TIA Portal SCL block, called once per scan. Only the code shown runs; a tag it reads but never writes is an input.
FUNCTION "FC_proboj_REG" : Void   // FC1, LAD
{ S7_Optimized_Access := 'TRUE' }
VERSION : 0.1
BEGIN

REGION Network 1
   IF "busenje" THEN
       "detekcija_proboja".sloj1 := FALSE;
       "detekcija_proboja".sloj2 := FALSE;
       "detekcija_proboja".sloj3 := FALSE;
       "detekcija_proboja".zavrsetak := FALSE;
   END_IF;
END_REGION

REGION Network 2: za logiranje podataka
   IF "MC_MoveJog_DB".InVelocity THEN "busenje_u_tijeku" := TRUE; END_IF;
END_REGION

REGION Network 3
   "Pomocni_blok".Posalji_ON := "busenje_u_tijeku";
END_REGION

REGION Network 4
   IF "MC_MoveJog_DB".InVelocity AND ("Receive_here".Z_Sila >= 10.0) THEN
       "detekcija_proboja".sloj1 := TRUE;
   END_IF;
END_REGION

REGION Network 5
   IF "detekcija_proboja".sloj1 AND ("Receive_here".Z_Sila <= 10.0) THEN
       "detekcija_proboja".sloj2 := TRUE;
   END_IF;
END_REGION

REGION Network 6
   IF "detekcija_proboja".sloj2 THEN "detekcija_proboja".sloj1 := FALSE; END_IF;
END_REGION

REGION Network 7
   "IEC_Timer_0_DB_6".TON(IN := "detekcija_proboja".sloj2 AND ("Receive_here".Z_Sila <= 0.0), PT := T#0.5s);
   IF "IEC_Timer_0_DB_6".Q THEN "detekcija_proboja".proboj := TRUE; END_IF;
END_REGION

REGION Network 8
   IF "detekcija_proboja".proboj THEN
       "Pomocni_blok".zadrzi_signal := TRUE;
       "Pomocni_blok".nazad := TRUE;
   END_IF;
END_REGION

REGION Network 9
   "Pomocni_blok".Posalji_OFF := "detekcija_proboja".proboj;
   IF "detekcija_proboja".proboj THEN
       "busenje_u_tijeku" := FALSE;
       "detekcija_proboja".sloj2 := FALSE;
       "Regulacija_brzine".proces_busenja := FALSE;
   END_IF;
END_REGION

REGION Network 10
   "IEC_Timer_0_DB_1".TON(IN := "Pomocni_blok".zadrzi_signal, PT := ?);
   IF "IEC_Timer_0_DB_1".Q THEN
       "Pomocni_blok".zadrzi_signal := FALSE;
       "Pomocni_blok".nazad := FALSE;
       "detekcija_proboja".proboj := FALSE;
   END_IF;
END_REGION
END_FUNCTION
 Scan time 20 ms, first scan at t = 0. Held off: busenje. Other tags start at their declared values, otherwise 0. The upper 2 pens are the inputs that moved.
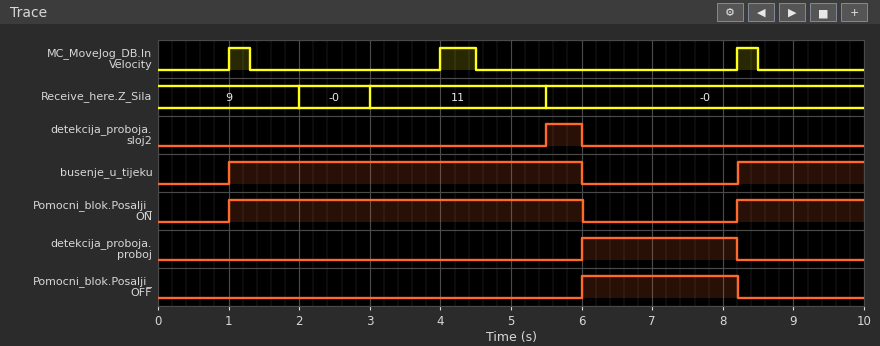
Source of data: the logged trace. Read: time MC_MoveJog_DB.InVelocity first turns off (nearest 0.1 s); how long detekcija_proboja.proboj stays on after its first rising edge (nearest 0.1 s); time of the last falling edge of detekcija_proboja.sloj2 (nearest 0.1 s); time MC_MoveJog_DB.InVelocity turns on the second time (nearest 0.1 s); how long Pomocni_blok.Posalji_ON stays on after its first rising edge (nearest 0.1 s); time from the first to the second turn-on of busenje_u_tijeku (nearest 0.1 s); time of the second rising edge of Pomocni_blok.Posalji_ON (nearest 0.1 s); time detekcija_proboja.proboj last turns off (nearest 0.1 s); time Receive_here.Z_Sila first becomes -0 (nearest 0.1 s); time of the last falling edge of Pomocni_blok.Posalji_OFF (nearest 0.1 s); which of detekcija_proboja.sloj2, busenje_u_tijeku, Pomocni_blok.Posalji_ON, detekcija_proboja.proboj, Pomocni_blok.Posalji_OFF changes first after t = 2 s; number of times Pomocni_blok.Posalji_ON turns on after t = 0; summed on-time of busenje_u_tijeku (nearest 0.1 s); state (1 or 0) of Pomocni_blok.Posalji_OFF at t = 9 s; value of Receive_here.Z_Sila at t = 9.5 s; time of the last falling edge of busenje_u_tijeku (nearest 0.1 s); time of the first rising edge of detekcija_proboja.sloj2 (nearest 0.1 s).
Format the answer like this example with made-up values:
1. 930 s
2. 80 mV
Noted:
1. 1.3 s
2. 2.2 s
3. 6.0 s
4. 4.0 s
5. 5.0 s
6. 7.2 s
7. 8.2 s
8. 8.2 s
9. 2.0 s
10. 8.2 s
11. detekcija_proboja.sloj2
12. 2
13. 6.8 s
14. 0
15. -0
16. 6.0 s
17. 5.5 s
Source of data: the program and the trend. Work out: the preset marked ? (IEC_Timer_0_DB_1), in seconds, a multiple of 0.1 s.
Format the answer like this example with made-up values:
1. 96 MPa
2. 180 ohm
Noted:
1. 2.2 s
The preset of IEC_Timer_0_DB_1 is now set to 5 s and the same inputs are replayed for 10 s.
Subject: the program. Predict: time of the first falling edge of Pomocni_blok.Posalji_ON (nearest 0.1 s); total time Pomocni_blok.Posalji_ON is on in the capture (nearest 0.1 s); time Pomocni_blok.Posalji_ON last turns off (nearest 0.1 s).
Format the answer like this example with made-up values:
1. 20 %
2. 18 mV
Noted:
1. 6.0 s
2. 5.3 s
3. 8.5 s
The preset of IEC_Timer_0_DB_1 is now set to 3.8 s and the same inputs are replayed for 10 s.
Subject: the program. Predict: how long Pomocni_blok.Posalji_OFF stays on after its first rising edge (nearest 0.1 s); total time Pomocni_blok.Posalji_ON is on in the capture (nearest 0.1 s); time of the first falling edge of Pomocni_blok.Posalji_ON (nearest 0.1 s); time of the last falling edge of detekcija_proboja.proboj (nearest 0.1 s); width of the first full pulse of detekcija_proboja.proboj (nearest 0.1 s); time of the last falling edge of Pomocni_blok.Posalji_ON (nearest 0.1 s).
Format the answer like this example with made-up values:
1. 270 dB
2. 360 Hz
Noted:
1. 3.8 s
2. 5.3 s
3. 6.0 s
4. 9.8 s
5. 3.8 s
6. 8.5 s
